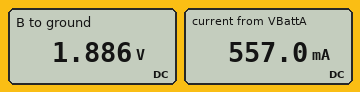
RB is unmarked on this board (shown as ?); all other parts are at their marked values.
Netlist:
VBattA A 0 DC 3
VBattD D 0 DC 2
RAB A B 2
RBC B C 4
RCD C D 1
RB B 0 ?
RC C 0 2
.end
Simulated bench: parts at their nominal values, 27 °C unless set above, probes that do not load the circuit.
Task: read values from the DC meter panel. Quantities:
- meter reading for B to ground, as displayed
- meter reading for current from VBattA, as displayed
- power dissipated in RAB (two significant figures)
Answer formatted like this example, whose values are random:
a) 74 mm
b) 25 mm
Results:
a) 1.886 V
b) 557.0 mA
c) 620 mW
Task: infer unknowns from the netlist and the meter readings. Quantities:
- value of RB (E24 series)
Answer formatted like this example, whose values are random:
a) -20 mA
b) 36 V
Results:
a) 4.3 Ω
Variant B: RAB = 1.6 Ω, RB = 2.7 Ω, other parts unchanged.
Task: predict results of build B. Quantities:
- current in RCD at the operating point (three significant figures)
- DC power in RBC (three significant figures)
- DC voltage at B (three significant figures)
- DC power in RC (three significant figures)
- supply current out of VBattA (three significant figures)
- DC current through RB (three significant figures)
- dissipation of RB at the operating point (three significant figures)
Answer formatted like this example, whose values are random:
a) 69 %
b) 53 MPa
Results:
a) 602 mA
b) 37.7 mW
c) 1.79 V
d) 977 mW
e) 759 mA
f) 662 mA
g) 1.18 W
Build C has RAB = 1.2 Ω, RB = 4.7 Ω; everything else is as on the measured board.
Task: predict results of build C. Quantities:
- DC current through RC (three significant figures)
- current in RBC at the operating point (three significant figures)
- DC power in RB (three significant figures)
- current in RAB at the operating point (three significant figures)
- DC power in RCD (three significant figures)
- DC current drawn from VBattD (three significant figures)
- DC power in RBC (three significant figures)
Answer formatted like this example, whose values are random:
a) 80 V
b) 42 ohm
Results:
a) 729 mA
b) 188 mA
c) 1.04 W
d) 658 mA
e) 293 mW
f) 541 mA
g) 141 mW
